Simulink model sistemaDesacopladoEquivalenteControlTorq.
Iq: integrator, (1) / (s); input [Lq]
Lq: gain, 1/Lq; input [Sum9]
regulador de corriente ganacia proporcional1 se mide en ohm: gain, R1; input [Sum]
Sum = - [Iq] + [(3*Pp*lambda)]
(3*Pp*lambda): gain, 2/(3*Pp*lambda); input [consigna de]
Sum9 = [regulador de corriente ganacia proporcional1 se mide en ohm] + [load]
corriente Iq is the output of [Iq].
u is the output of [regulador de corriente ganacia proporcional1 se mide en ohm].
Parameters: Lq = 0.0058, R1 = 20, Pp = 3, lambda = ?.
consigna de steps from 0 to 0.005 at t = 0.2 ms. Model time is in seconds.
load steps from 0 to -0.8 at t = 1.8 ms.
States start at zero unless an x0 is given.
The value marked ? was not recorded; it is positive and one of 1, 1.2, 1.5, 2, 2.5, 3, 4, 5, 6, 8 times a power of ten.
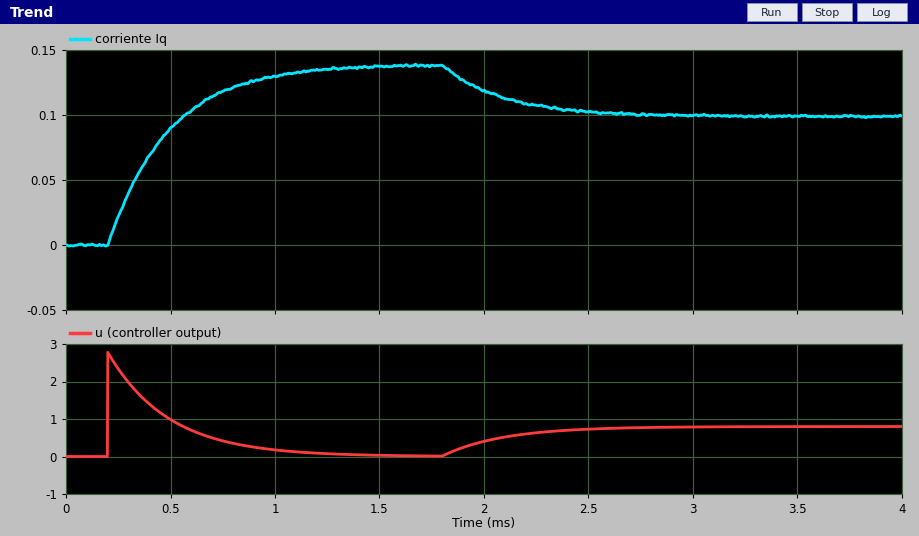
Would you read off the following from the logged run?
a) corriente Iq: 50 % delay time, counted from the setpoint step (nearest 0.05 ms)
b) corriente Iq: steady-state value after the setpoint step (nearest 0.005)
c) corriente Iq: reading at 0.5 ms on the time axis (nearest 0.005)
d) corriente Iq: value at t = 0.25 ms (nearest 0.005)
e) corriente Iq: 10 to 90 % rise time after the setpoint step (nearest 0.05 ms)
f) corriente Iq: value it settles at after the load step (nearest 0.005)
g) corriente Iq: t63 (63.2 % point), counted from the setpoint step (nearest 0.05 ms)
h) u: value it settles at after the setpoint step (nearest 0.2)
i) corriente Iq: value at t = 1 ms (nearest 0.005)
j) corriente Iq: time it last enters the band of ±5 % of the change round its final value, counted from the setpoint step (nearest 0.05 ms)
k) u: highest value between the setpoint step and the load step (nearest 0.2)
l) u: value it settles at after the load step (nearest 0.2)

0.20 ms
0.140
0.090
0.020
0.65 ms
0.100
0.30 ms
0.0
0.130
0.85 ms
2.8
0.8
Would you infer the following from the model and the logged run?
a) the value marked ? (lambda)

0.008
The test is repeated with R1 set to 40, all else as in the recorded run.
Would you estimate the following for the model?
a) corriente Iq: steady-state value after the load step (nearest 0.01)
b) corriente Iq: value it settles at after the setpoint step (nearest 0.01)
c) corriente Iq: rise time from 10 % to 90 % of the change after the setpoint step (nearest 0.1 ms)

0.12
0.14
0.3 ms
